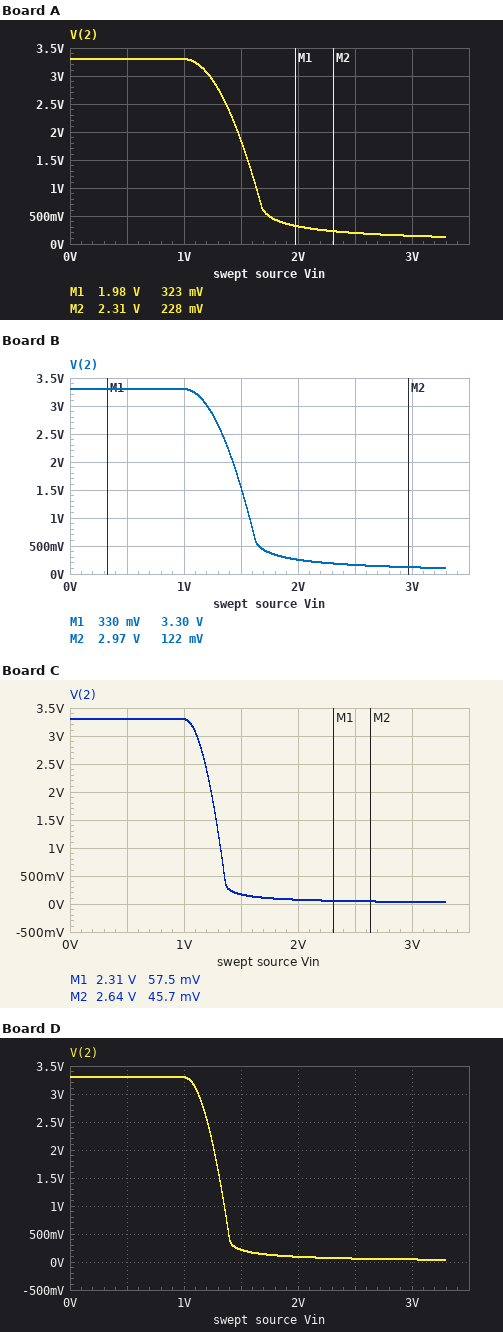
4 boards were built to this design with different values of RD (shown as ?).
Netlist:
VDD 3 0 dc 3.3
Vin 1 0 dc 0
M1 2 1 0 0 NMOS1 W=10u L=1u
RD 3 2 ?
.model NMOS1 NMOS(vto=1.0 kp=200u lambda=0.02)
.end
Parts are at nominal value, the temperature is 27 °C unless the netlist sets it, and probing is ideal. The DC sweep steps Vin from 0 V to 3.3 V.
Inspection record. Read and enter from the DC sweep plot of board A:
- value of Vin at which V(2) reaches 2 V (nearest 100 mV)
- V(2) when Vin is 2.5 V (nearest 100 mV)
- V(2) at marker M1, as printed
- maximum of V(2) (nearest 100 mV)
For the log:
1.5 V
200 mV
323 mV
3.3 V
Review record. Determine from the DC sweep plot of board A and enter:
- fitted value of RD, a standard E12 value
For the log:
5.6 kΩ
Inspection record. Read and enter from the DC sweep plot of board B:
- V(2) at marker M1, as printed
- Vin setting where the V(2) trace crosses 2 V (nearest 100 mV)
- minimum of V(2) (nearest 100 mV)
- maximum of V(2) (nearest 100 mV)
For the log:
3.30 V
1.4 V
100 mV
3.3 V
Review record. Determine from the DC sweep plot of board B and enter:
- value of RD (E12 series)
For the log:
6.8 kΩ
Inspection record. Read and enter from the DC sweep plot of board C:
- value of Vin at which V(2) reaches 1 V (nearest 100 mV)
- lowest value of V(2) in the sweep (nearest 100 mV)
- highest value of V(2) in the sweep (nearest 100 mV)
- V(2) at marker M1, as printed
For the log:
1.3 V
0 V
3.3 V
57.5 mV
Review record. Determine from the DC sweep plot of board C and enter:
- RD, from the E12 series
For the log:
22 kΩ
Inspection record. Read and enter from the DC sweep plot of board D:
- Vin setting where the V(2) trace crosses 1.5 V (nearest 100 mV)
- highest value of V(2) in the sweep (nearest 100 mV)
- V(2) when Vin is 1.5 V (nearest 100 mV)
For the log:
1.3 V
3.3 V
200 mV
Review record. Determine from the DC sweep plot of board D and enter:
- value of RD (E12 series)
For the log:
18 kΩ
